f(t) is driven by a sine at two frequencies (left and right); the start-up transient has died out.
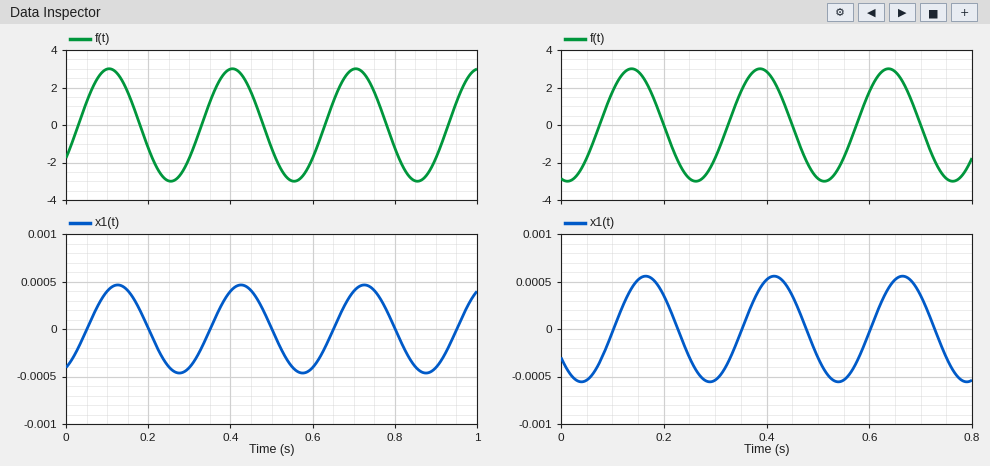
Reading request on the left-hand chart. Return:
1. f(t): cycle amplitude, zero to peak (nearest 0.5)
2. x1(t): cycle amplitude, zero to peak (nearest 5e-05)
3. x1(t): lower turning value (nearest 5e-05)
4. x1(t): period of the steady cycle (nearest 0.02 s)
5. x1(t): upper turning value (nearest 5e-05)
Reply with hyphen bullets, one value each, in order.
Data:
- 3.0
- 0.00045
- -0.00045
- 0.30 s
- 0.00045
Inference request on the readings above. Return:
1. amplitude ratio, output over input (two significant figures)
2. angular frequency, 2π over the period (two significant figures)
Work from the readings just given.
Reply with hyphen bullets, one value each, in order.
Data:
- 0.00015
- 21 rad/s
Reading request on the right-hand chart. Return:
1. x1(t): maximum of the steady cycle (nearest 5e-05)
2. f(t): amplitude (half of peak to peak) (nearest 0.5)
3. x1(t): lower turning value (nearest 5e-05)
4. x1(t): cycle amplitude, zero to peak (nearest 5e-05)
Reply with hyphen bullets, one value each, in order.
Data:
- 0.00055
- 3.0
- -0.00055
- 0.00055
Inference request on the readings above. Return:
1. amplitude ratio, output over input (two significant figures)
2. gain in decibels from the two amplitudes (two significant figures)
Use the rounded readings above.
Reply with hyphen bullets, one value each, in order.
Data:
- 0.00018
- -75 dB
